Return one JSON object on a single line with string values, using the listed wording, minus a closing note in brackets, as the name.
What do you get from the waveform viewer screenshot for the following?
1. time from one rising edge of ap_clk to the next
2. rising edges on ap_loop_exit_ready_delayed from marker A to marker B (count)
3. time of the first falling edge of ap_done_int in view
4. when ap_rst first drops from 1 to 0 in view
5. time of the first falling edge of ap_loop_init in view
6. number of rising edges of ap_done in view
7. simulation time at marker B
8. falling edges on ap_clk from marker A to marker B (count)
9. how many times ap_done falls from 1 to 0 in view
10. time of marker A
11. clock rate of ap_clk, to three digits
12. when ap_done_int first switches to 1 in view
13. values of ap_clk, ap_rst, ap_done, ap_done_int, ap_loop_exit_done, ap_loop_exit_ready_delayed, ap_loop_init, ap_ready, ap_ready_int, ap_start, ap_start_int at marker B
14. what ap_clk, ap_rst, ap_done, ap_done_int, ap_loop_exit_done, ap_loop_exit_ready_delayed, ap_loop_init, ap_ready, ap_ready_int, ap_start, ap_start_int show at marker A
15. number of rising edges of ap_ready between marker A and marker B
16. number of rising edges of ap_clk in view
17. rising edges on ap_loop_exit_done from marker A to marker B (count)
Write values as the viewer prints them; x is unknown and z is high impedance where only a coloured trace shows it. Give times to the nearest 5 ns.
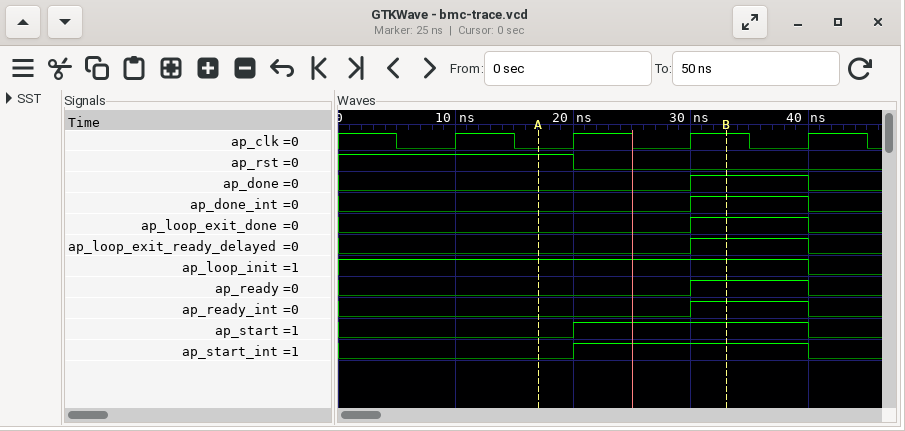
{"time from one rising edge of ap_clk to the next": "10 ns", "rising edges on ap_loop_exit_ready_delayed from marker A to marker B": "1", "time of the first falling edge of ap_done_int in view": "40 ns", "when ap_rst first drops from 1 to 0 in view": "20 ns", "time of the first falling edge of ap_loop_init in view": "40 ns", "number of rising edges of ap_done in view": "1", "simulation time at marker B": "35 ns", "falling edges on ap_clk from marker A to marker B": "1", "how many times ap_done falls from 1 to 0 in view": "1", "time of marker A": "15 ns", "clock rate of ap_clk, to three digits": "100 MHz", "when ap_done_int first switches to 1 in view": "30 ns", "values of ap_clk, ap_rst, ap_done, ap_done_int, ap_loop_exit_done, ap_loop_exit_ready_delayed, ap_loop_init, ap_ready, ap_ready_int, ap_start, ap_start_int at marker B": "ap_clk=1, ap_rst=0, ap_done=1, ap_done_int=1, ap_loop_exit_done=1, ap_loop_exit_ready_delayed=1, ap_loop_init=1, ap_ready=1, ap_ready_int=1, ap_start=1, ap_start_int=1", "what ap_clk, ap_rst, ap_done, ap_done_int, ap_loop_exit_done, ap_loop_exit_ready_delayed, ap_loop_init, ap_ready, ap_ready_int, ap_start, ap_start_int show at marker A": "ap_clk=0, ap_rst=1, ap_done=0, ap_done_int=0, ap_loop_exit_done=0, ap_loop_exit_ready_delayed=0, ap_loop_init=1, ap_ready=0, ap_ready_int=0, ap_start=0, ap_start_int=0", "number of rising edges of ap_ready between marker A and marker B": "1", "number of rising edges of ap_clk in view": "4", "rising edges on ap_loop_exit_done from marker A to marker B": "1"}
